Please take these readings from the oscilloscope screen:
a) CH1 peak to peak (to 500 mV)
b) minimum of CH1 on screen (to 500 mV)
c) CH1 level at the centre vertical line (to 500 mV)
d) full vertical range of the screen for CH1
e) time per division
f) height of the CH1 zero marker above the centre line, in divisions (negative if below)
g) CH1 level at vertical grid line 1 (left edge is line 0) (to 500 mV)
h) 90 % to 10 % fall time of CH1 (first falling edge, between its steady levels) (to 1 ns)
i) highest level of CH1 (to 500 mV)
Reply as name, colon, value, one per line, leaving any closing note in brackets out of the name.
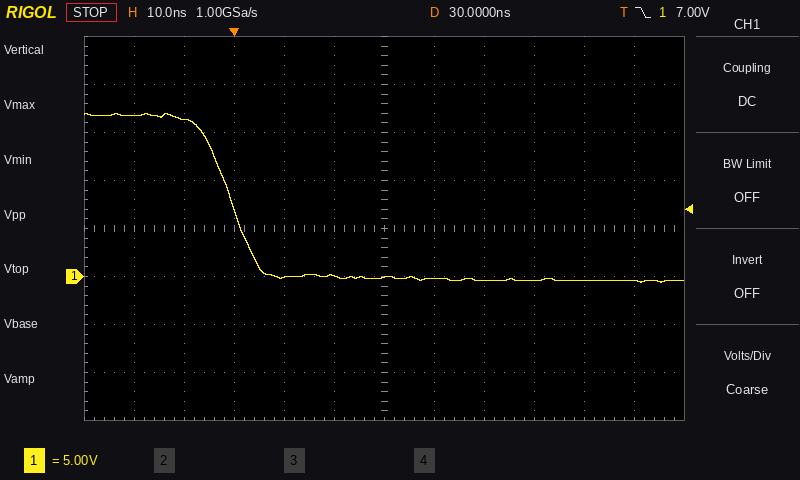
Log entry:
CH1 peak to peak: 17.5 V
minimum of CH1 on screen: -500 mV
CH1 level at the centre vertical line: 0.0 V
full vertical range of the screen for CH1: 40 V
time per division: 10 ns
height of the CH1 zero marker above the centre line, in divisions: -1.0 div
CH1 level at vertical grid line 1 (left edge is line 0): 17.0 V
90 % to 10 % fall time of CH1 (first falling edge, between its steady levels): 11 ns
highest level of CH1: 17.0 V
